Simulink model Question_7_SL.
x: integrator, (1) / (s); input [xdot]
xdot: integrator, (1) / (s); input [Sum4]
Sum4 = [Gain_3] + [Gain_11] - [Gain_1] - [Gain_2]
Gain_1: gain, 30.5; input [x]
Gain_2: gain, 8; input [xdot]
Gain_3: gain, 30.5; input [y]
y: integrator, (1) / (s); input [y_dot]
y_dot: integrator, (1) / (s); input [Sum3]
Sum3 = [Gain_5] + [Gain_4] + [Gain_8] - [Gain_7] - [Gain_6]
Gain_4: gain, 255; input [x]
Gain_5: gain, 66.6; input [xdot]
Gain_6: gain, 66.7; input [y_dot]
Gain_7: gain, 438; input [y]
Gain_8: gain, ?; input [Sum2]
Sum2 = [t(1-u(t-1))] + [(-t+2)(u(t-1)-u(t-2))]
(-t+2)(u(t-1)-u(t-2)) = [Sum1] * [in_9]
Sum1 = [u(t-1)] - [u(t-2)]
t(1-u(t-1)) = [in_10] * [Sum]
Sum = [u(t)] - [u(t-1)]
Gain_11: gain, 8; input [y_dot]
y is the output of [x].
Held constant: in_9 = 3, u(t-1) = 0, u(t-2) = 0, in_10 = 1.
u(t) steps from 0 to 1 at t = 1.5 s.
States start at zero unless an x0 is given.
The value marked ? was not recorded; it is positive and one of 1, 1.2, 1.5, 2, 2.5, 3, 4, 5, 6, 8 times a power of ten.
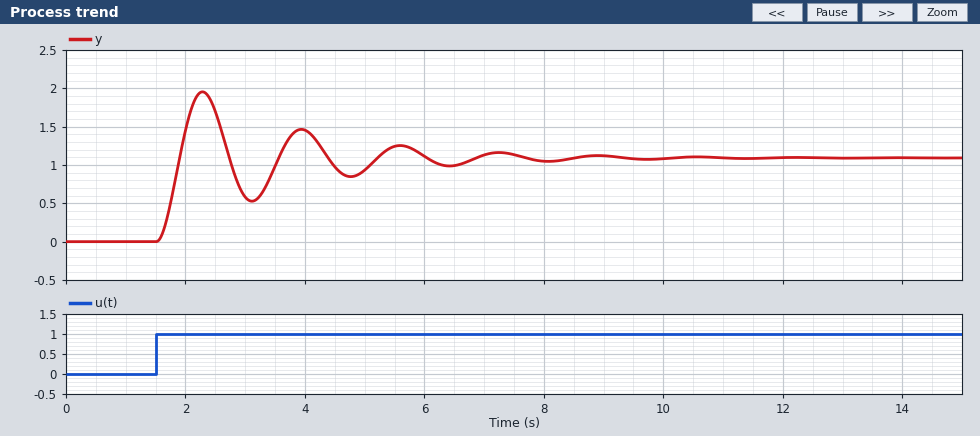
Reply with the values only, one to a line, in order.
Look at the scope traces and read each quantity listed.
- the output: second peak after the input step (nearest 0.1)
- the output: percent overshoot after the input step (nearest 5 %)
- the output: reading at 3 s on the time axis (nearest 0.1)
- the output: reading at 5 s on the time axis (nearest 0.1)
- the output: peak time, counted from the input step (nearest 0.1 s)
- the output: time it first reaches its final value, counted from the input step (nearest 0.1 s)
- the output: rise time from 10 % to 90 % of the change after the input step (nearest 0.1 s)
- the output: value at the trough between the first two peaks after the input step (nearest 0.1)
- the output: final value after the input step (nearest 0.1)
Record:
1.5
80 %
0.6
0.9
0.8 s
0.4 s
0.3 s
0.5
1.1
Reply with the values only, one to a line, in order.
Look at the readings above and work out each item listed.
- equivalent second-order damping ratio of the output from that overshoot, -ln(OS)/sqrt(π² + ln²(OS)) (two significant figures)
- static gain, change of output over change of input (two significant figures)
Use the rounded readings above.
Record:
0.071
1.1
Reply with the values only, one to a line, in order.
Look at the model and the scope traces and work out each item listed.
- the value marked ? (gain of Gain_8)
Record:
200
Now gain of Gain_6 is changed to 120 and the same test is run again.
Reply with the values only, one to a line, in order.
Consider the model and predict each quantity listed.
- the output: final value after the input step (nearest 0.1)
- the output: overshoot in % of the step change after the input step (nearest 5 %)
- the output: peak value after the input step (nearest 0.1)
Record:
1.1
15 %
1.3
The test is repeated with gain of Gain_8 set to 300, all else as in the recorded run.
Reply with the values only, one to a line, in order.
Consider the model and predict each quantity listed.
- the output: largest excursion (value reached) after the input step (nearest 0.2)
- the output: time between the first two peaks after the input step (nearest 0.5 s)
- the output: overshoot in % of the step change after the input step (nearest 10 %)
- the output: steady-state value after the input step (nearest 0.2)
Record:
3.0
1.5 s
80 %
1.6
